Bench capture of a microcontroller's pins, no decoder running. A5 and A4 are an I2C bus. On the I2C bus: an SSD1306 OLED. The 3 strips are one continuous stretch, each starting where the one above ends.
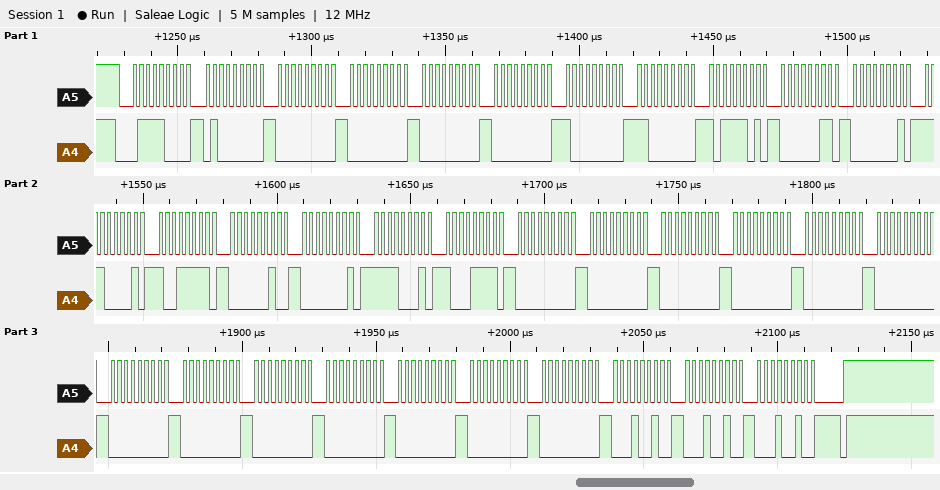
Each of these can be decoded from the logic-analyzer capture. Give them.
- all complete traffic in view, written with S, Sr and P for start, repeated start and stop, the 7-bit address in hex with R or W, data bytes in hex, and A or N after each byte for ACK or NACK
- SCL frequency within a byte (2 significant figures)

S 3CW A 40 A 00 A 00 A 00 A 00 A 80 A C0 A BD A 03 A 01 A E1 A 9F A 02 A 01 A F1 A 8F A 00 A 00 A 00 A 00 A 00 A 00 A 00 A 00 A 00 A 00 A 00 A 00 A 00 A 12 A 12 A 12 A P
400 kHz
